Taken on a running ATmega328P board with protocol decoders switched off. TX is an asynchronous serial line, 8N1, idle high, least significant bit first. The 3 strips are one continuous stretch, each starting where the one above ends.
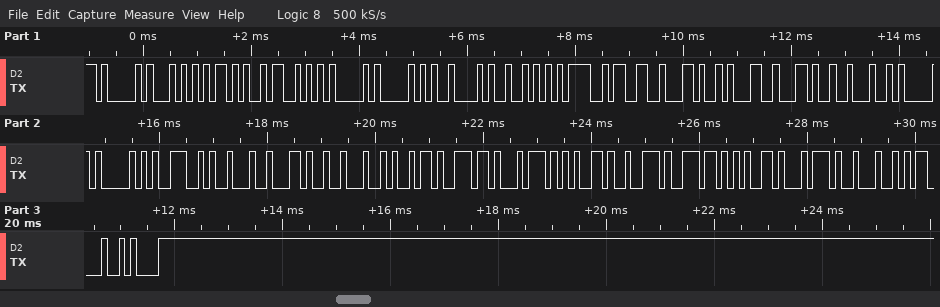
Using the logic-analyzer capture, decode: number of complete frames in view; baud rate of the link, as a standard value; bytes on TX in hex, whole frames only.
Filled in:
31
9600 baud
41 54 2B 53 41 50 42 52 3D 33 2C 31 2C 22 41 50 4E 22 2C 22 69 6E 74 65 72 6E 65 74 22 0D 0A
